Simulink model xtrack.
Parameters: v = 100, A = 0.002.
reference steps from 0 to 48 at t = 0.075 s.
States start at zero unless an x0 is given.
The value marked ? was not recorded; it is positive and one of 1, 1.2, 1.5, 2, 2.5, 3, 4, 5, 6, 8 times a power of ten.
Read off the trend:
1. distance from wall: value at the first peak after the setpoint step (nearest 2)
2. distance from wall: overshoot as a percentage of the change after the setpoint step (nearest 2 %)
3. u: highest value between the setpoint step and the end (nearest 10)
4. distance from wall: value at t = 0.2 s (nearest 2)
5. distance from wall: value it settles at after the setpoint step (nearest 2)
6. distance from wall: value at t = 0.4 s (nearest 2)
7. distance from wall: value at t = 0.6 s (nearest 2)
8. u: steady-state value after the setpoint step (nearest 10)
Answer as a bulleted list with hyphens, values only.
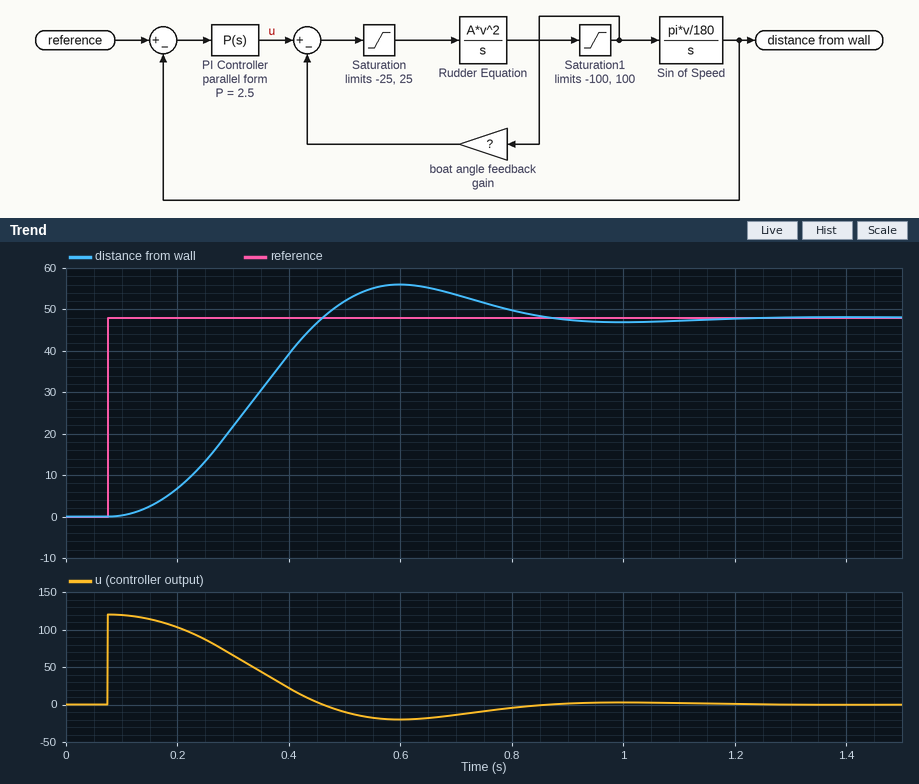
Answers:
- 56
- 16 %
- 120
- 6
- 48
- 40
- 56
- 0
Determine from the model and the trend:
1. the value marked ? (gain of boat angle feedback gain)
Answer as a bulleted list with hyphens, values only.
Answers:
- 0.5
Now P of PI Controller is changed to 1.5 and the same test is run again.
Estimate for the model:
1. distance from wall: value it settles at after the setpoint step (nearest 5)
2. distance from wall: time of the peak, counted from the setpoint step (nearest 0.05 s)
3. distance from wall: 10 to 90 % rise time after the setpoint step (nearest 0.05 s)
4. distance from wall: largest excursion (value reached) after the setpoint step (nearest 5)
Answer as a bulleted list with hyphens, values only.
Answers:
- 50
- 0.65 s
- 0.30 s
- 50
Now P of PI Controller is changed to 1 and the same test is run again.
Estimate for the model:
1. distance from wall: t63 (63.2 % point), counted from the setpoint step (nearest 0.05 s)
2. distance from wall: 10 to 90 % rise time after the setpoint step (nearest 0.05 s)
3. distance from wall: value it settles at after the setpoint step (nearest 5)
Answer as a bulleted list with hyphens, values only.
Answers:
- 0.35 s
- 0.45 s
- 50
